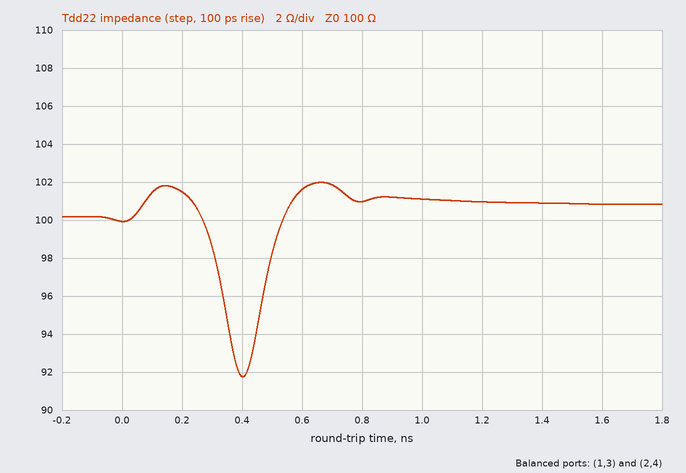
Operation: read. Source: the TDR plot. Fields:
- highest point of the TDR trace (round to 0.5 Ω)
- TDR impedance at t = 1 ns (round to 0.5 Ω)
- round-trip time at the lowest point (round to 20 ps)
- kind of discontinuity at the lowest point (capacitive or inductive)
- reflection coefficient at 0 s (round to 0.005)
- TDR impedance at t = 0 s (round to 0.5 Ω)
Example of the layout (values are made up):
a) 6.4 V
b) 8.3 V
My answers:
a) 102.0 Ω
b) 101.0 Ω
c) 400 ps
d) capacitive
e) 0.000
f) 100.0 Ω
